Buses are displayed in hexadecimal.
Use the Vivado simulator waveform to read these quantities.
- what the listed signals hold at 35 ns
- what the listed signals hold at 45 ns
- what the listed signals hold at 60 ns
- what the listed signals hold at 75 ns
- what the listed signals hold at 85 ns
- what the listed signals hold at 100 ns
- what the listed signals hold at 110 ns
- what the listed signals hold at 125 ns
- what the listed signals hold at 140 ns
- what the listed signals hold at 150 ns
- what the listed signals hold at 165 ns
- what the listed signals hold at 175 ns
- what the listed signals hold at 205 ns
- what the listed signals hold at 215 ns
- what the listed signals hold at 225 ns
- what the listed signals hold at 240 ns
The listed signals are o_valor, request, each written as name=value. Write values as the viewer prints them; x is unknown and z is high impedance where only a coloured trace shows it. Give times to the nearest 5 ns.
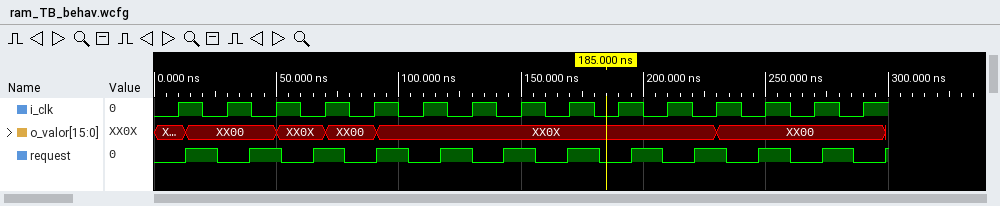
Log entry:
o_valor=XX00, request=0
o_valor=XX00, request=1
o_valor=XX0X, request=0
o_valor=XX00, request=1
o_valor=XX00, request=0
o_valor=XX0X, request=1
o_valor=XX0X, request=0
o_valor=XX0X, request=1
o_valor=XX0X, request=0
o_valor=XX0X, request=1
o_valor=XX0X, request=0
o_valor=XX0X, request=1
o_valor=XX0X, request=1
o_valor=XX0X, request=0
o_valor=XX0X, request=1
o_valor=XX00, request=0
